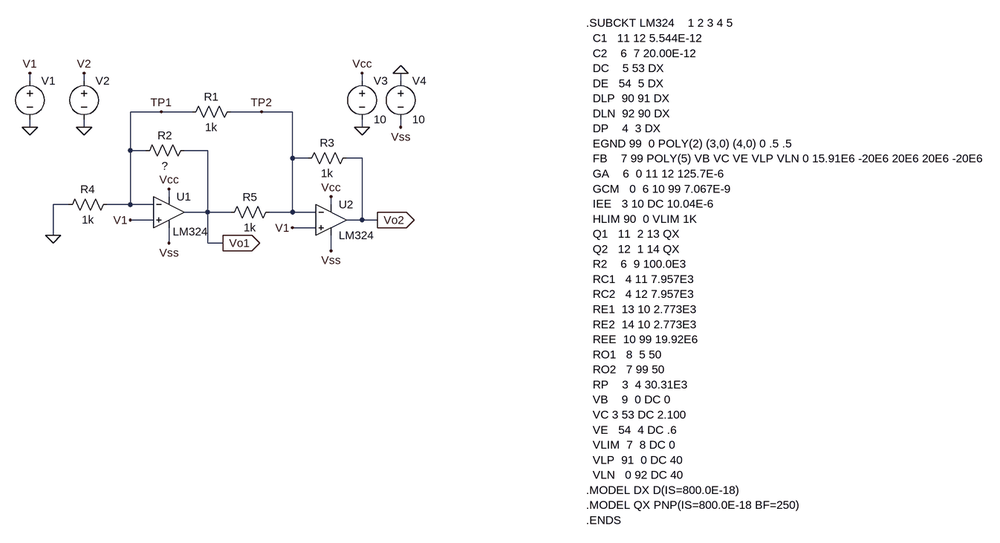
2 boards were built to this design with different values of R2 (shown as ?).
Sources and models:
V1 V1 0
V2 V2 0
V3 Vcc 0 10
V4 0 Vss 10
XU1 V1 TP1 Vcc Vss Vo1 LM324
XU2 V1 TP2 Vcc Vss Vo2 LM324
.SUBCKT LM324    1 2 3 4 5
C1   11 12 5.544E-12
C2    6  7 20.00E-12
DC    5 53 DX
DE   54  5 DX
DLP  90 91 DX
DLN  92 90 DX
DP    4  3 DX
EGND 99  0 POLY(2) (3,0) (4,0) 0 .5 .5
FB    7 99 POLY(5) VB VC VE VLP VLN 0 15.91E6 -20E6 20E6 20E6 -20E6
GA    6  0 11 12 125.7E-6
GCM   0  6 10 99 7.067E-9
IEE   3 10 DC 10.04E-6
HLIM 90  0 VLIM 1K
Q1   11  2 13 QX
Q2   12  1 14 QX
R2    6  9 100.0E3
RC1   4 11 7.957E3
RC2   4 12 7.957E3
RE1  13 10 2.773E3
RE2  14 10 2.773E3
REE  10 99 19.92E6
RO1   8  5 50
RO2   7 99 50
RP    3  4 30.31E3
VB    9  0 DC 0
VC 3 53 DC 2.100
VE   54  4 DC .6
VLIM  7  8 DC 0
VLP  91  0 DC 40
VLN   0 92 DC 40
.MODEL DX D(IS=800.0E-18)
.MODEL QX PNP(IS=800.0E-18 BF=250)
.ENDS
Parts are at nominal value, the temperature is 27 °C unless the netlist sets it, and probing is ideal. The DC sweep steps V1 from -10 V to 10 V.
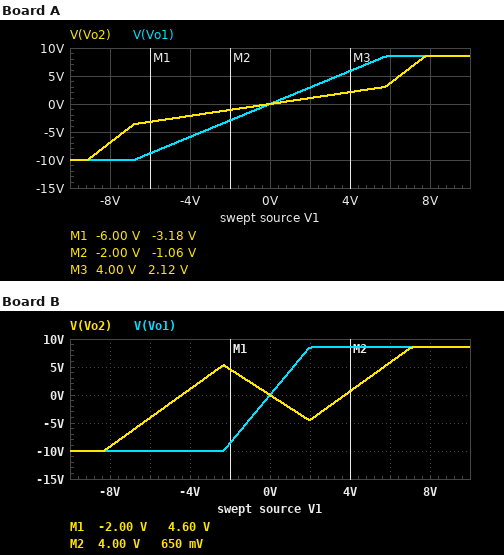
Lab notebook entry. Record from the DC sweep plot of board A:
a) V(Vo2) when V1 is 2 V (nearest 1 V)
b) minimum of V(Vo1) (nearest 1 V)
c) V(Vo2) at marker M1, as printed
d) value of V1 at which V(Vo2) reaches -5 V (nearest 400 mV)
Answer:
1 V
-10 V
-3.18 V
-7.2 V
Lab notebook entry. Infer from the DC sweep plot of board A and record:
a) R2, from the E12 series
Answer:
470 Ω
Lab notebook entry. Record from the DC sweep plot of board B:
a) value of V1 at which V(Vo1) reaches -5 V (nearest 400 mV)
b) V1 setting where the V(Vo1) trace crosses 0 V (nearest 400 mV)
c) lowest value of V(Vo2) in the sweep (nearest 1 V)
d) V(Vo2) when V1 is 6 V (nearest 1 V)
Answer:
-1.2 V
0 V
-10 V
6 V
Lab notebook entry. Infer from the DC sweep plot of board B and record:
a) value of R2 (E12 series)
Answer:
3.3 kΩ
